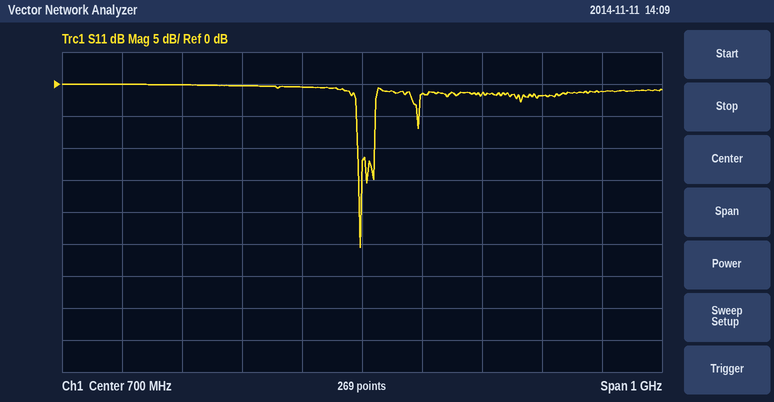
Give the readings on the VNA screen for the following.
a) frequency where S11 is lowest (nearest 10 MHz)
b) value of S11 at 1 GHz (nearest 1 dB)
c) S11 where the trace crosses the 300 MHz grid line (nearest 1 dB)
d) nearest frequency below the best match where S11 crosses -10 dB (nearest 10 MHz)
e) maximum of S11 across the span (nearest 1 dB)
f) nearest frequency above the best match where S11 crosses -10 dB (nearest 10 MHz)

700 MHz
-2 dB
0 dB
690 MHz
0 dB
720 MHz
